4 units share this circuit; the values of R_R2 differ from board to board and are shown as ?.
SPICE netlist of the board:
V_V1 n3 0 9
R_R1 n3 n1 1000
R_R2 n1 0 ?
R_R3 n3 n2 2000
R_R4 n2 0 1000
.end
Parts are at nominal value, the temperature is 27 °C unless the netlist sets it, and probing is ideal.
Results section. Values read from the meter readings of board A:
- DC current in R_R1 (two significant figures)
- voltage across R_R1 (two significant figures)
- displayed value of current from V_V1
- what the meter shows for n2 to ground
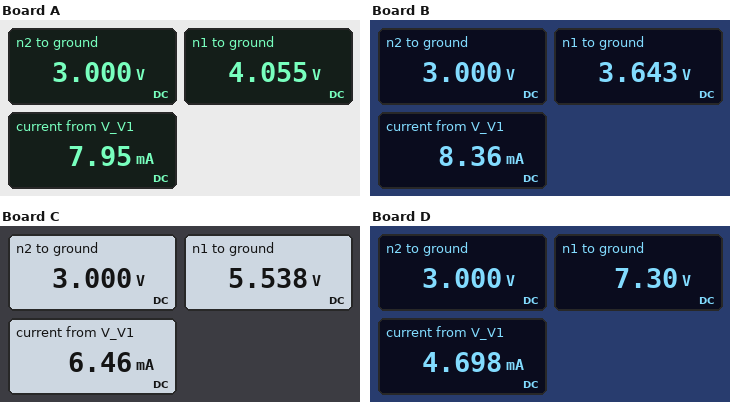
4.9 mA
4.9 V
7.95 mA
3.000 V
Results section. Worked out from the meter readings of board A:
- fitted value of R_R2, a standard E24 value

820 Ω
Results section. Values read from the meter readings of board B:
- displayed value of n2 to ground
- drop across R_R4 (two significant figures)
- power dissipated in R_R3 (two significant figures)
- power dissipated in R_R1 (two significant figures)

3.000 V
3.0 V
18 mW
29 mW
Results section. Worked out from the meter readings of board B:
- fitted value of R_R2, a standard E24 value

680 Ω
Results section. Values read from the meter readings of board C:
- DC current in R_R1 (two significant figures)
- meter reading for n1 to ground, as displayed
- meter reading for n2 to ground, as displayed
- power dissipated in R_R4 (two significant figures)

3.5 mA
5.538 V
3.000 V
9.0 mW
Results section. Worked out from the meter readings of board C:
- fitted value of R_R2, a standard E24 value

1.6 kΩ
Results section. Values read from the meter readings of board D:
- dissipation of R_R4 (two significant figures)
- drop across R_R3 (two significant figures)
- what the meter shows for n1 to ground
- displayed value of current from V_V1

9.0 mW
6.0 V
7.30 V
4.698 mA
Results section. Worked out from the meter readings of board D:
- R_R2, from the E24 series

4.3 kΩ
